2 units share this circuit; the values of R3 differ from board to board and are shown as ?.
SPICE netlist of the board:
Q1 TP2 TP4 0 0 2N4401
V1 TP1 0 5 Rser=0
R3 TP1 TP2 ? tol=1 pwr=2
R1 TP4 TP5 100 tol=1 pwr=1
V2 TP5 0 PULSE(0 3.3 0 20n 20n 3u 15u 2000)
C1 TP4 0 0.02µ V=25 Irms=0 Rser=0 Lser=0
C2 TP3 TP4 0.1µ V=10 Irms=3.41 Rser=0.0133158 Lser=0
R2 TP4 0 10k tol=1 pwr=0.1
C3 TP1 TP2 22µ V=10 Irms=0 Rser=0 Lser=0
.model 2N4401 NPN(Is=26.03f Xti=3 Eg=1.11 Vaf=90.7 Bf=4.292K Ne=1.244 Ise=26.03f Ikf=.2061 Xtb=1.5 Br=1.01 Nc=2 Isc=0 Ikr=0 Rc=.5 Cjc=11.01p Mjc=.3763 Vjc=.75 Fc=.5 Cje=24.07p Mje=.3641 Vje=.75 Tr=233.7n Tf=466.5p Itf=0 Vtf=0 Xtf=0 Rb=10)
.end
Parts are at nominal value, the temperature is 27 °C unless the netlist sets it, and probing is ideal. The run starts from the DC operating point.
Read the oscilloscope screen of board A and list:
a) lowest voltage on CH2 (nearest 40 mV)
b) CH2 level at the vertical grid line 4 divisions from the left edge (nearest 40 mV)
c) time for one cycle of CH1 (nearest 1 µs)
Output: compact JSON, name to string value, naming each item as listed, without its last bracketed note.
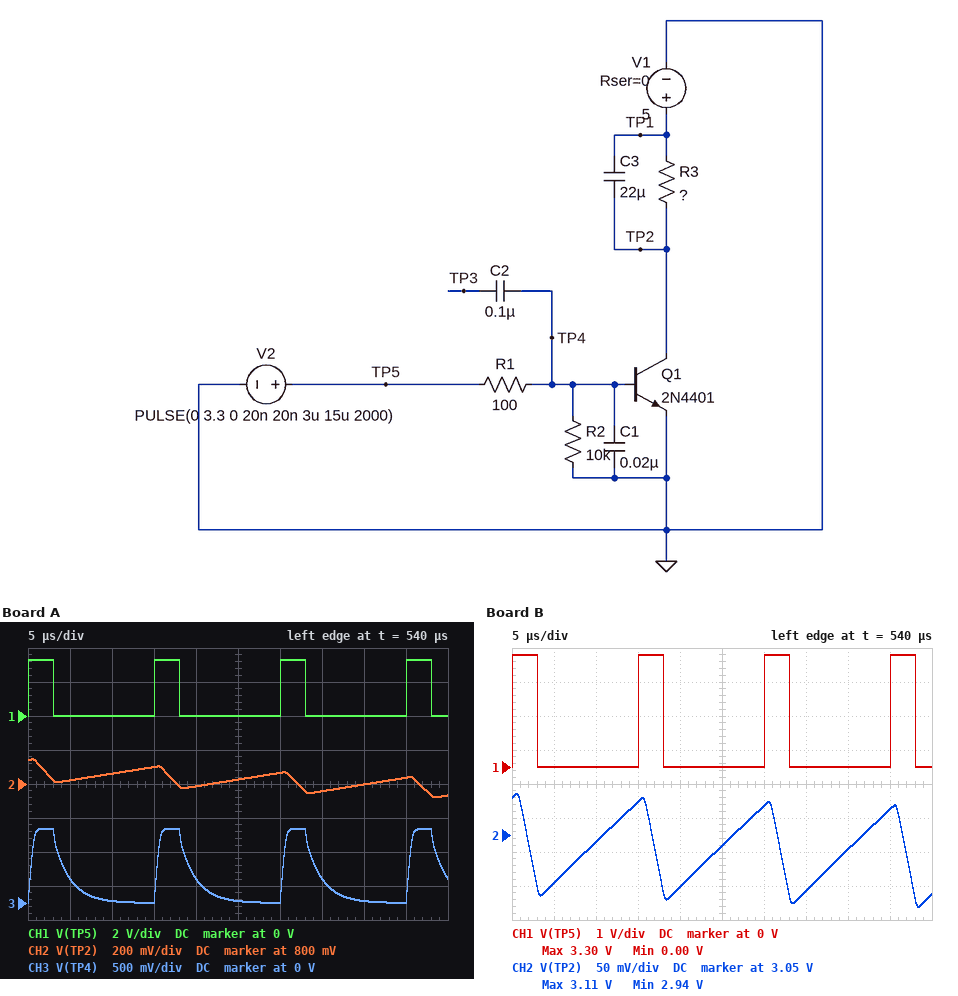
{"lowest voltage on CH2": "720 mV", "CH2 level at the vertical grid line 4 divisions from the left edge": "800 mV", "time for one cycle of CH1": "15 µs"}
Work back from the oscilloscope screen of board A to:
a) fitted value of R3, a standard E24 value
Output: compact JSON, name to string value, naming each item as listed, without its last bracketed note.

{"fitted value of R3, a standard E24 value": "24 Ω"}
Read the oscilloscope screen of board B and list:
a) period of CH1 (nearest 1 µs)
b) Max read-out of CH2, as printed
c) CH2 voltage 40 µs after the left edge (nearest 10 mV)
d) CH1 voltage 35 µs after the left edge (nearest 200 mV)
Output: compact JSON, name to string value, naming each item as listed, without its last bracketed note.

{"period of CH1": "15 µs", "Max read-out of CH2, as printed": "3.11 V", "CH2 voltage 40 µs after the left edge": "3.03 V", "CH1 voltage 35 µs after the left edge": "0 V"}
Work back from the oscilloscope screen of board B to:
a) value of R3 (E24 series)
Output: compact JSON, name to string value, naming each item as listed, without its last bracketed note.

{"value of R3": "7.5 Ω"}
